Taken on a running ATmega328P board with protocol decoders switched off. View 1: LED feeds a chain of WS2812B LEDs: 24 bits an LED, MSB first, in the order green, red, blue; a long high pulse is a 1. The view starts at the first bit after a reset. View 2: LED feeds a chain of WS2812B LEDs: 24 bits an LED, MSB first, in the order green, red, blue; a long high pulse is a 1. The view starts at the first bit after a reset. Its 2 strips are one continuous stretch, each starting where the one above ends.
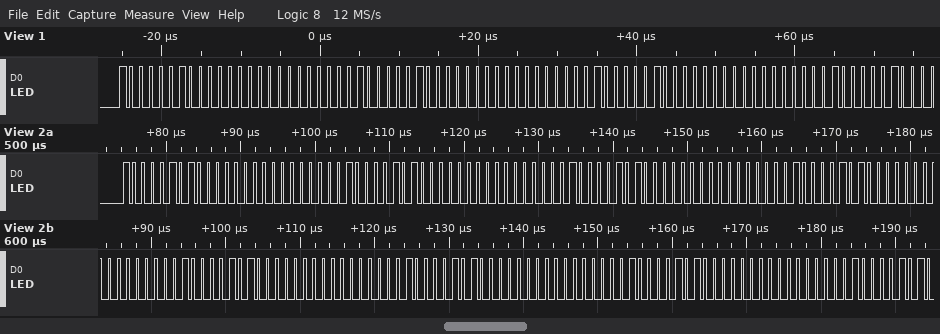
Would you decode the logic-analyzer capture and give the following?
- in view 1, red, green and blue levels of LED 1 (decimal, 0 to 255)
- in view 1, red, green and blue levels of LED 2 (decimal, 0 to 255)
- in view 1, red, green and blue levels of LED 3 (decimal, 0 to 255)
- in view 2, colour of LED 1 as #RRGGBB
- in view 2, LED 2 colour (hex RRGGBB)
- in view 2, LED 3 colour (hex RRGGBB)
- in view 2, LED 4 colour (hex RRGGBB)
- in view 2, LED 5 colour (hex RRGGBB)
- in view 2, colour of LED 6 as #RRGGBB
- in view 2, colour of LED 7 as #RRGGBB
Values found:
0, 130, 0
0, 130, 0
0, 130, 0
#008500
#008500
#008500
#008500
#008500
#008500
#008500
